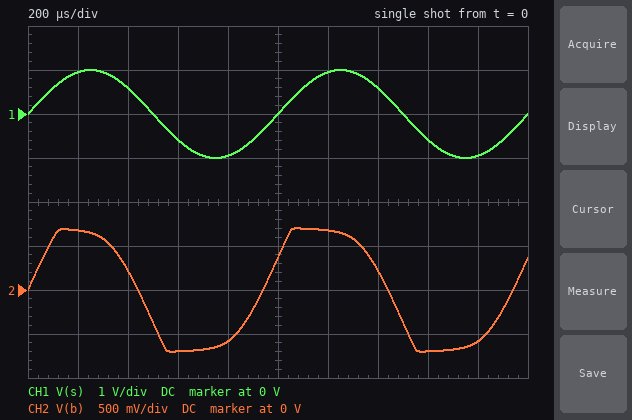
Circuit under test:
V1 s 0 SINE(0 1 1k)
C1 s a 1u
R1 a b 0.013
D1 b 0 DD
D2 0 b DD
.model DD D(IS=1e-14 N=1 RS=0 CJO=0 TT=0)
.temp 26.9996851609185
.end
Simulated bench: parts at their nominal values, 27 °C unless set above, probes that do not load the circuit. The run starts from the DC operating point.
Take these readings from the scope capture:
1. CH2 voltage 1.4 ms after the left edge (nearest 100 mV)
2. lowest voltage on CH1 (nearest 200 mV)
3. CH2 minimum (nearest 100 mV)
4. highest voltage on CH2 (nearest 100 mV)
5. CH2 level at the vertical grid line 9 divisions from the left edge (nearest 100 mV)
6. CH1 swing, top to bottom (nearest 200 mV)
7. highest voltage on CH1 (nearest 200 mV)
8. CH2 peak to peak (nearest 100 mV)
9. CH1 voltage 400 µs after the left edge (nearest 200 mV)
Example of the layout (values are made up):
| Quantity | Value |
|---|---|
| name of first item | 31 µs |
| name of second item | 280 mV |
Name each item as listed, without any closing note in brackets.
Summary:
| Quantity | Value |
|---|---|
| CH2 voltage 1.4 ms after the left edge | 200 mV |
| lowest voltage on CH1 | -1.0 V |
| CH2 minimum | -700 mV |
| highest voltage on CH2 | 700 mV |
| CH2 level at the vertical grid line 9 divisions from the left edge | -600 mV |
| CH1 swing, top to bottom | 2.0 V |
| highest voltage on CH1 | 1.0 V |
| CH2 peak to peak | 1.4 V |
| CH1 voltage 400 µs after the left edge | 600 mV |
